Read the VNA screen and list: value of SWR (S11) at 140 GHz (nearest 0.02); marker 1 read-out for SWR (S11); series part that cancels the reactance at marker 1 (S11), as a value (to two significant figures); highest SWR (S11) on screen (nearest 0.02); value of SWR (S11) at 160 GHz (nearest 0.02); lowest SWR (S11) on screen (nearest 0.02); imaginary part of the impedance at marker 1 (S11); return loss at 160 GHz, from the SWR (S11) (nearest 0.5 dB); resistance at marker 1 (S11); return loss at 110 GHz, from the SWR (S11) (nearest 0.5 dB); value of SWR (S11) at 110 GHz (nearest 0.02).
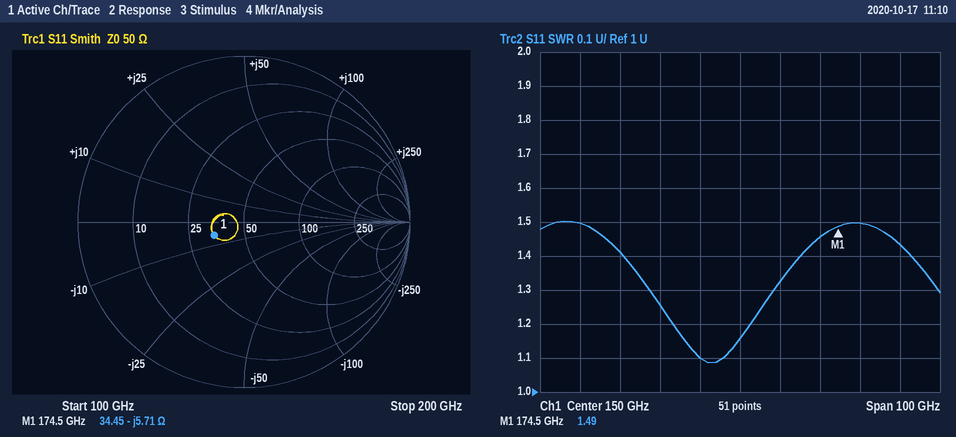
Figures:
1.10
1.49
5.2 pH
1.50
1.32
1.08
-5.71 Ω
17.0 dB
34.45 Ω
14.0 dB
1.50
